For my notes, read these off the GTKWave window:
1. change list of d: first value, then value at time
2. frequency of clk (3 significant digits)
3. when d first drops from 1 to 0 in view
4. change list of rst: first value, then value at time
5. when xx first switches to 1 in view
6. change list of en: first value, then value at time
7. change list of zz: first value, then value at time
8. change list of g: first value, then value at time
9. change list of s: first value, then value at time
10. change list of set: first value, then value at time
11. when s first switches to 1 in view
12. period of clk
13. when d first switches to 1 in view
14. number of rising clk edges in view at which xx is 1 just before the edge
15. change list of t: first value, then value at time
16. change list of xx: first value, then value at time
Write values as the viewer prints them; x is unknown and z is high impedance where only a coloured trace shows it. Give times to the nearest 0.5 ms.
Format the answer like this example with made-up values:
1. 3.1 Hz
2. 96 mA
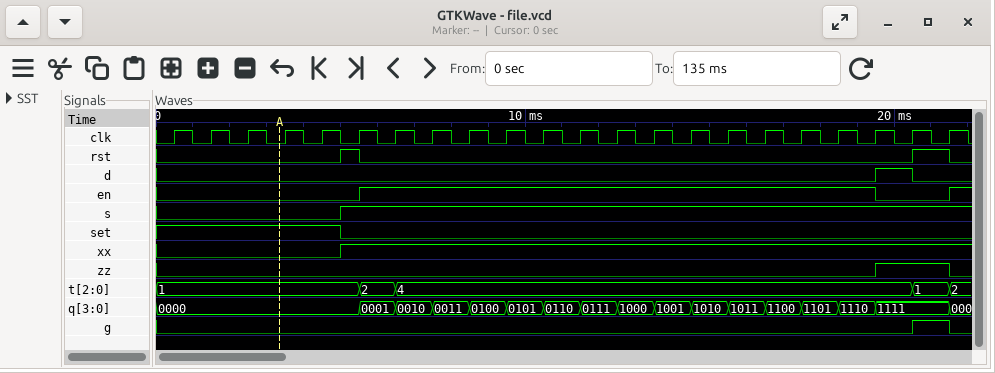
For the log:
1. 0, 1 at 19.5 ms, 0 at 20.5 ms
2. 1.00 kHz
3. 20.5 ms
4. 0, 1 at 5 ms, 0 at 5.5 ms, 1 at 20.5 ms, 0 at 21.5 ms
5. 5 ms
6. 0, 1 at 5.5 ms, 0 at 19.5 ms, 1 at 21.5 ms
7. 0, 1 at 19.5 ms, 0 at 21.5 ms
8. 0, 1 at 20.5 ms, 0 at 21.5 ms
9. 0, 1 at 5 ms
10. 1, 0 at 5 ms
11. 5 ms
12. 1 ms
13. 19.5 ms
14. 17
15. 1, 2 at 5.5 ms, 4 at 6.5 ms, 1 at 20.5 ms, 2 at 21.5 ms
16. 0, 1 at 5 ms
